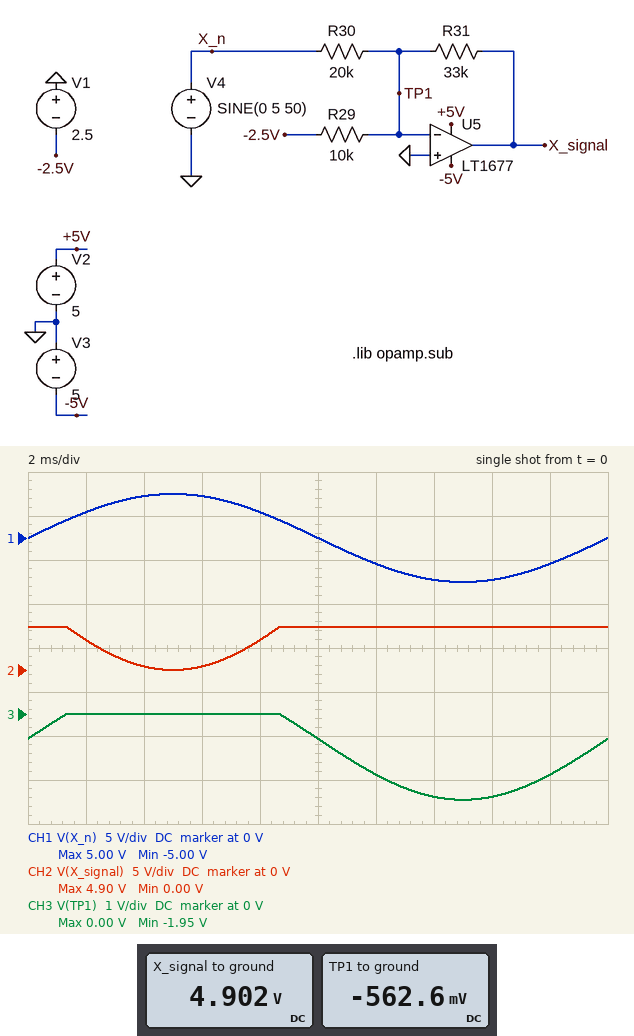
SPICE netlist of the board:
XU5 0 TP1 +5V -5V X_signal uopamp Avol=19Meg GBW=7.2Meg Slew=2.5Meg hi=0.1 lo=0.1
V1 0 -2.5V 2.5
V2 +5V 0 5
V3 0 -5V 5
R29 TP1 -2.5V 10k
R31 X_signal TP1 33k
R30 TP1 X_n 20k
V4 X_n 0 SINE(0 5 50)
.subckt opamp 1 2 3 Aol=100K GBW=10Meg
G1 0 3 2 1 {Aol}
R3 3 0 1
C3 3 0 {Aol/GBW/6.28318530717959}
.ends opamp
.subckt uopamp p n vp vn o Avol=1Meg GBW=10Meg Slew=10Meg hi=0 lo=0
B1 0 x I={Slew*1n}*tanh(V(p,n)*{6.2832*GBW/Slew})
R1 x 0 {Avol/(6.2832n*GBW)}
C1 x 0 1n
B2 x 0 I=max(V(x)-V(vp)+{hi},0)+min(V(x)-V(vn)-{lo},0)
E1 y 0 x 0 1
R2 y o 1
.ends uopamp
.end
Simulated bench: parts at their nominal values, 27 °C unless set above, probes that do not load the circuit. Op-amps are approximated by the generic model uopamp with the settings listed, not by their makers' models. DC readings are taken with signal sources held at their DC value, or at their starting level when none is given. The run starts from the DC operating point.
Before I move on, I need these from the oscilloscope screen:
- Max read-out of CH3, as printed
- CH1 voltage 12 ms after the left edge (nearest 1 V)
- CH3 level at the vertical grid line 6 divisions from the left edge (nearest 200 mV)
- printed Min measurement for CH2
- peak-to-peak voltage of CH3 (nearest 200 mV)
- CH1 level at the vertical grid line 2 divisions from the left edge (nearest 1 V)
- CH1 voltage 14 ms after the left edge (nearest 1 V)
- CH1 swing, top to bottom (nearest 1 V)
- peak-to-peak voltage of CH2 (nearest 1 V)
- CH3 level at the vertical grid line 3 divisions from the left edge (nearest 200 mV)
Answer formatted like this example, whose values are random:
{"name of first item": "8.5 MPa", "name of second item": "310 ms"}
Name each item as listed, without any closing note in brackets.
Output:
{"Max read-out of CH3, as printed": "0.00 V", "CH1 voltage 12 ms after the left edge": "-3 V", "CH3 level at the vertical grid line 6 divisions from the left edge": "-1.4 V", "printed Min measurement for CH2": "0.00 V", "peak-to-peak voltage of CH3": "2.0 V", "CH1 level at the vertical grid line 2 divisions from the left edge": "5 V", "CH1 voltage 14 ms after the left edge": "-5 V", "CH1 swing, top to bottom": "10 V", "peak-to-peak voltage of CH2": "5 V", "CH3 level at the vertical grid line 3 divisions from the left edge": "0 V"}
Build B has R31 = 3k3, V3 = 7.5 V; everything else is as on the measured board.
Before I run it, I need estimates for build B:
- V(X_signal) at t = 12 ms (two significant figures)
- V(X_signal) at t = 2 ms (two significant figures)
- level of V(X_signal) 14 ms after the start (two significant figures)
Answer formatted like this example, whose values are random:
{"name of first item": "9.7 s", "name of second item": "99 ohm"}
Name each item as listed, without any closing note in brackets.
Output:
{"V(X_signal) at t = 12 ms": "1.3 V", "V(X_signal) at t = 2 ms": "340 mV", "level of V(X_signal) 14 ms after the start": "1.6 V"}
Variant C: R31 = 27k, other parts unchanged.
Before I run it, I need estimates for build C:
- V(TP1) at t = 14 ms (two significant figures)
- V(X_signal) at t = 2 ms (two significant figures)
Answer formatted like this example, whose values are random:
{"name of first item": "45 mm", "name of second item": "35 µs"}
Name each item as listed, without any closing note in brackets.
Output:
{"V(TP1) at t = 14 ms": "-1.6 V", "V(X_signal) at t = 2 ms": "2.8 V"}
